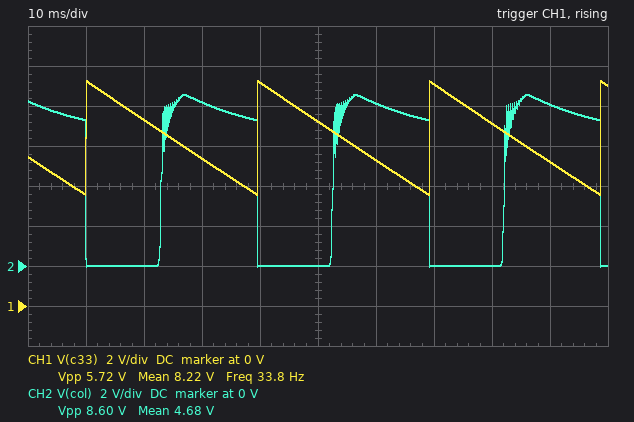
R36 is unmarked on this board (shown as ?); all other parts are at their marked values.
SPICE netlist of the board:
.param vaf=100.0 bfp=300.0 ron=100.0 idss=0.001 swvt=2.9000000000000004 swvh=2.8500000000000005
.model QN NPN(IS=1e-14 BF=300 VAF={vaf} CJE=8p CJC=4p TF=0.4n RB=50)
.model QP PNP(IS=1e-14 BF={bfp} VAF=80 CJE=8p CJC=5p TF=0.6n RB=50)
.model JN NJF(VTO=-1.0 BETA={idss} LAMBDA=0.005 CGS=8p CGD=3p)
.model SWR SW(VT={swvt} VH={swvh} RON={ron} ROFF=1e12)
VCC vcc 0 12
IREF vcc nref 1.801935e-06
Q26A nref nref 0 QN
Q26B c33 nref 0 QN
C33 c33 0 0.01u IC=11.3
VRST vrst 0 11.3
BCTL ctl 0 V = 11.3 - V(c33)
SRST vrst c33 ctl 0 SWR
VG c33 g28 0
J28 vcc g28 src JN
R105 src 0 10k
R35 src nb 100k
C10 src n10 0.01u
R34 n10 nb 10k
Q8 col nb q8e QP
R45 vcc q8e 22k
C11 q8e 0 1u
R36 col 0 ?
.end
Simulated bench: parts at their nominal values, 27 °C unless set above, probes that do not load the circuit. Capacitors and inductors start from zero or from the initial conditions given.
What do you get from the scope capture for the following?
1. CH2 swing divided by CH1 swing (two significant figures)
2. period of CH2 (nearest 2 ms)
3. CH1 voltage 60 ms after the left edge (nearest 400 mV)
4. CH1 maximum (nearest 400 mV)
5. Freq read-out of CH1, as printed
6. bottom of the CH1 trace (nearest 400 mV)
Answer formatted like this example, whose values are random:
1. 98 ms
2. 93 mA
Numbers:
1. 1.5
2. 30 ms
3. 7.2 V
4. 11.2 V
5. 33.8 Hz
6. 5.6 V
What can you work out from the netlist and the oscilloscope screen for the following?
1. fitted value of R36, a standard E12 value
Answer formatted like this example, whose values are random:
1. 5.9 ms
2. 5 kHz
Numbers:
1. 27 kΩ
